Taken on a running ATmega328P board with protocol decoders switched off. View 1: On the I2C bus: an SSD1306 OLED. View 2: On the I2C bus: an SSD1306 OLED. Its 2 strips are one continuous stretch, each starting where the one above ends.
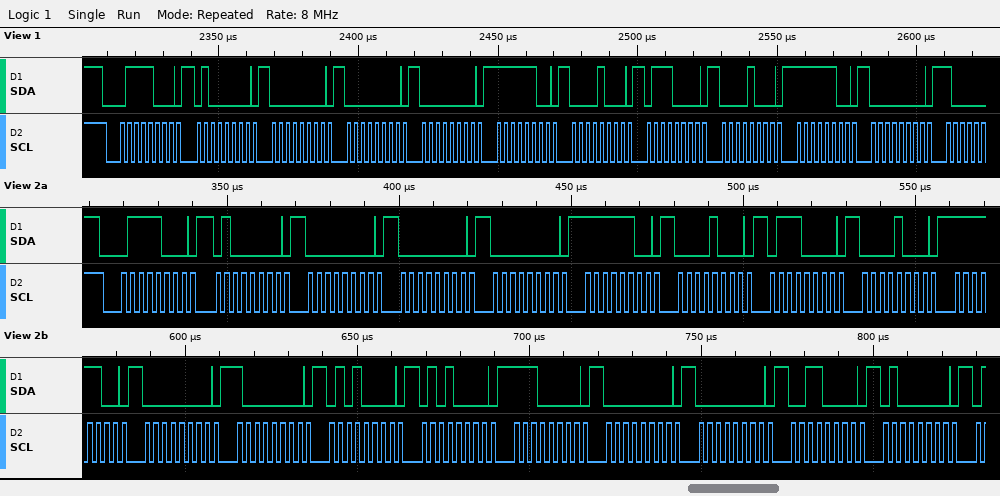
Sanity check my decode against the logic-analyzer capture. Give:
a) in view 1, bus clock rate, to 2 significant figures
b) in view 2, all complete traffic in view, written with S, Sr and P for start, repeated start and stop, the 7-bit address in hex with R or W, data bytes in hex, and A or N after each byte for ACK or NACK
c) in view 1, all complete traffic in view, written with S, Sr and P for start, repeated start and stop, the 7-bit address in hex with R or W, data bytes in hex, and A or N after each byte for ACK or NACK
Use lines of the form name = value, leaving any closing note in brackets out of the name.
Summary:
in view 1, bus clock rate, to 2 significant figures = 400 kHz
in view 2, all complete traffic in view, written with S, Sr and P for start, repeated start and stop, the 7-bit address in hex with R or W, data bytes in hex, and A or N after each byte for ACK or NACK = S 3CW A 40 A 00 A 00 A 00 A FC A 08 A 70 A 08 A FC A 00 A 80 A 50 A 50 A E0 A 00 A 00 A 30 A 40 A
in view 1, all complete traffic in view, written with S, Sr and P for start, repeated start and stop, the 7-bit address in hex with R or W, data bytes in hex, and A or N after each byte for ACK or NACK = S 3CW A 40 A 00 A 00 A 00 A FC A 08 A 70 A 08 A FC A 00 A
